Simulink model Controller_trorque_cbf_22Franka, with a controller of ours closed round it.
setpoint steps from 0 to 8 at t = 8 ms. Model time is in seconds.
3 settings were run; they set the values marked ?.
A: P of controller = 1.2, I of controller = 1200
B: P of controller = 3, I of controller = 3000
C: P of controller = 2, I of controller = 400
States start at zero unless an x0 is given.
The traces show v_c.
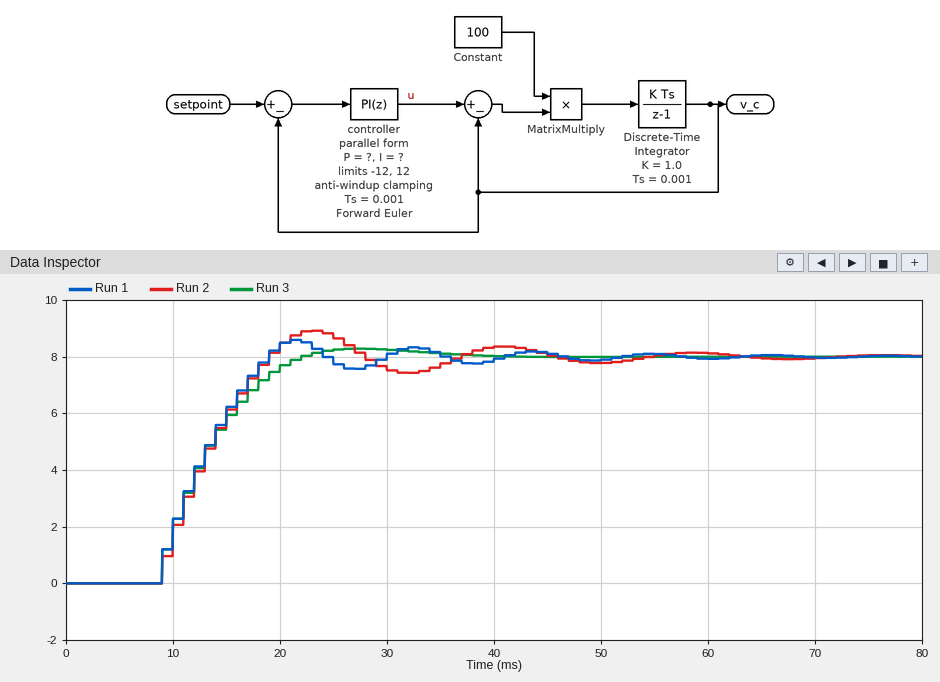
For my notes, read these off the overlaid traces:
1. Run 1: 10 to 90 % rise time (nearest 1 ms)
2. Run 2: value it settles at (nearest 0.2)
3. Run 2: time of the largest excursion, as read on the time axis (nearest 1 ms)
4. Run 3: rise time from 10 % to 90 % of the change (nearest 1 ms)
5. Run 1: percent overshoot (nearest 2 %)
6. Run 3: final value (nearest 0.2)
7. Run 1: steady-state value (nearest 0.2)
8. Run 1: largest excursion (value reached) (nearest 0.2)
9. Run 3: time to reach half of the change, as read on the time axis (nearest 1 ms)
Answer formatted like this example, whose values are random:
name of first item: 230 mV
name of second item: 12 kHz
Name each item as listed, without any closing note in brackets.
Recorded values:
Run 1: 10 to 90 % rise time: 8 ms
Run 2: value it settles at: 8.0
Run 2: time of the largest excursion, as read on the time axis: 23 ms
Run 3: rise time from 10 % to 90 % of the change: 10 ms
Run 1: percent overshoot: 8 %
Run 3: final value: 8.0
Run 1: steady-state value: 8.0
Run 1: largest excursion (value reached): 8.6
Run 3: time to reach half of the change, as read on the time axis: 12 ms
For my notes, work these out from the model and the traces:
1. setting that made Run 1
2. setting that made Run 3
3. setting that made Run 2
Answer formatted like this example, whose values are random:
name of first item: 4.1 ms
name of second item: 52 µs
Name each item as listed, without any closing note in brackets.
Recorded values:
setting that made Run 1: B
setting that made Run 3: C
setting that made Run 2: A
